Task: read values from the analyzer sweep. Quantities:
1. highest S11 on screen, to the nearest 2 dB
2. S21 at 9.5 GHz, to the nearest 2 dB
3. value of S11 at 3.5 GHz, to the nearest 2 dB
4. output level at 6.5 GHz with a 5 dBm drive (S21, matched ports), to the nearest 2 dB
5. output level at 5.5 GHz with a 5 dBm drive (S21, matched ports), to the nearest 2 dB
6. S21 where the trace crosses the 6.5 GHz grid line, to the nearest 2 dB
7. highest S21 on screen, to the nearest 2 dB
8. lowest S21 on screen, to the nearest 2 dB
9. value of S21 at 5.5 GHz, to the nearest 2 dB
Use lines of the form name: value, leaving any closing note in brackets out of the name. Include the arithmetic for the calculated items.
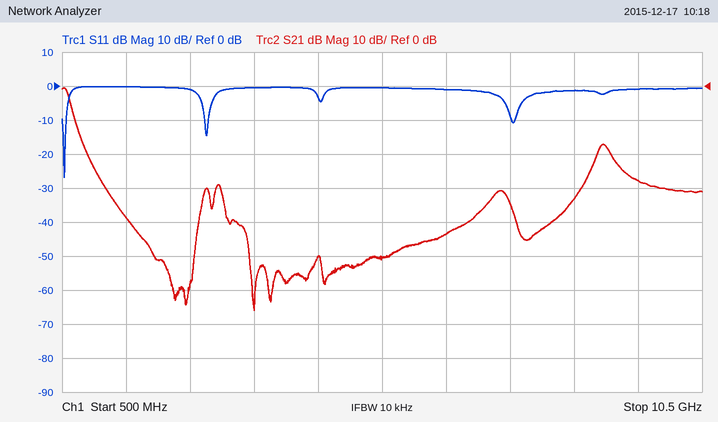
highest S11 on screen, to the nearest 2 dB: 0 dB
S21 at 9.5 GHz, to the nearest 2 dB: -28 dB
value of S11 at 3.5 GHz, to the nearest 2 dB: 0 dB
output level at 6.5 GHz with a 5 dBm drive (S21, matched ports), to the nearest 2 dB: 5 dBm + (-44 dB) = -38 dBm
output level at 5.5 GHz with a 5 dBm drive (S21, matched ports), to the nearest 2 dB: 5 dBm + (-50 dB) = -46 dBm
S21 where the trace crosses the 6.5 GHz grid line, to the nearest 2 dB: -44 dB
highest S21 on screen, to the nearest 2 dB: 0 dB
lowest S21 on screen, to the nearest 2 dB: -66 dB
value of S21 at 5.5 GHz, to the nearest 2 dB: -50 dB
